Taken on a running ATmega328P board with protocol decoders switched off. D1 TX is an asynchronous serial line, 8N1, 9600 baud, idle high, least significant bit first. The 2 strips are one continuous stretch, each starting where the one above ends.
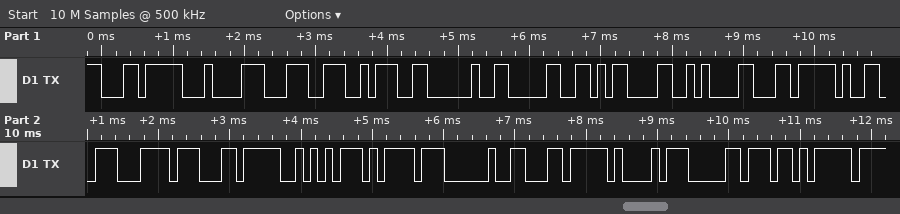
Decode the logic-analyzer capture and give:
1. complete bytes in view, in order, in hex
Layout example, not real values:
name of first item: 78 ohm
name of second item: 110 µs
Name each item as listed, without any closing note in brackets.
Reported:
complete bytes in view, in order, in hex: EC 84 9C 3A 20 30 0D 0A EC 99 BC EC AA BD 20 EC A1 B0 EB
